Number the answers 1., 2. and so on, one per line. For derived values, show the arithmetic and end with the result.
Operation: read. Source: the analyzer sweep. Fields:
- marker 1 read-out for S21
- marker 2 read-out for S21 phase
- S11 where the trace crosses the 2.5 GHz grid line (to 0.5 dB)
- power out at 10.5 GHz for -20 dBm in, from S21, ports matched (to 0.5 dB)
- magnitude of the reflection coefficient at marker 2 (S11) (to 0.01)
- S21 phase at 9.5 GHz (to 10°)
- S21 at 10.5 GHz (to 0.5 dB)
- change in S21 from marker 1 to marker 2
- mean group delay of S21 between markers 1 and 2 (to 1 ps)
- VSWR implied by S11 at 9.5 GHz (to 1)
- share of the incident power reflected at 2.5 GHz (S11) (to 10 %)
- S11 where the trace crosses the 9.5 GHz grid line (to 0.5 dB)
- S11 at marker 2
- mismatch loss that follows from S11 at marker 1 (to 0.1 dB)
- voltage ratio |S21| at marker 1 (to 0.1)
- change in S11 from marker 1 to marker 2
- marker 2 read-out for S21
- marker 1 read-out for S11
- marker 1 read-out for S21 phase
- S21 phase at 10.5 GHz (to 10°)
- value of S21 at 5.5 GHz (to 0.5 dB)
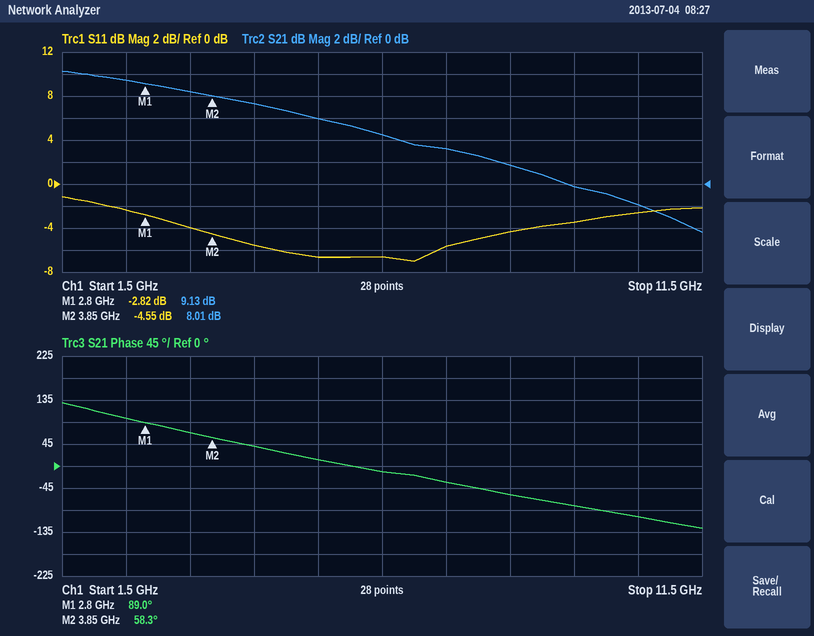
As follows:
1. 9.13 dB
2. 58.3°
3. -2.5 dB
4. -20 dBm + (-2.0 dB) = -22.0 dBm
5. 10^(-4.55/20) ≈ 0.59
6. -80°
7. -2.0 dB
8. 8.01 − (9.13) = -1.12 dB
9. −(58.3° − (89°))/(360° × 1.05 GHz) ≈ 81 ps
10. |Γ| = 10^(-3.5/20) = 0.6683; VSWR = (1 + 0.6683)/(1 − 0.6683) ≈ 5
11. 10^(-2.5/10) ≈ 56.2 %, so 60 % to the nearest 10 %
12. -3.5 dB
13. -4.55 dB
14. −10 log10(1 − 10^(-2.82/10)) ≈ 3.2 dB
15. 10^(9.13/20) ≈ 2.9
16. -4.55 − (-2.82) = -1.73 dB
17. 8.01 dB
18. -2.82 dB
19. 89.0°
20. -100°
21. 6.0 dB
